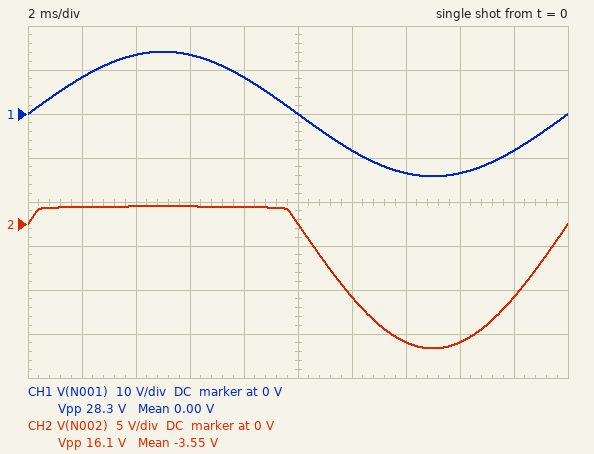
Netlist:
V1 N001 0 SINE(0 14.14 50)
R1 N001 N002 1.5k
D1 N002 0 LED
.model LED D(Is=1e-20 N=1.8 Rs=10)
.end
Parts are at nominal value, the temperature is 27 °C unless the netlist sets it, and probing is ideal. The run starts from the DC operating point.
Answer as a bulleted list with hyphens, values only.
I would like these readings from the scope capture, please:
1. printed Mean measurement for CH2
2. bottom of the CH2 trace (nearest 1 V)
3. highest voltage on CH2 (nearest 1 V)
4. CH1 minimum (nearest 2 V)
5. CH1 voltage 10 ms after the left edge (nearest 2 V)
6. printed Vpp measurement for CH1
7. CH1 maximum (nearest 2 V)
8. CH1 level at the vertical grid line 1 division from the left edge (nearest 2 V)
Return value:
- -3.55 V
- -14 V
- 2 V
- -14 V
- 0 V
- 28.3 V
- 14 V
- 8 V
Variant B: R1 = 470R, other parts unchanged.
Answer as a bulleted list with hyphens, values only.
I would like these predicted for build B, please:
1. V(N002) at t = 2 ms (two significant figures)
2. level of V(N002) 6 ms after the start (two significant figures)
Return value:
- 2.1 V
- 2.2 V
